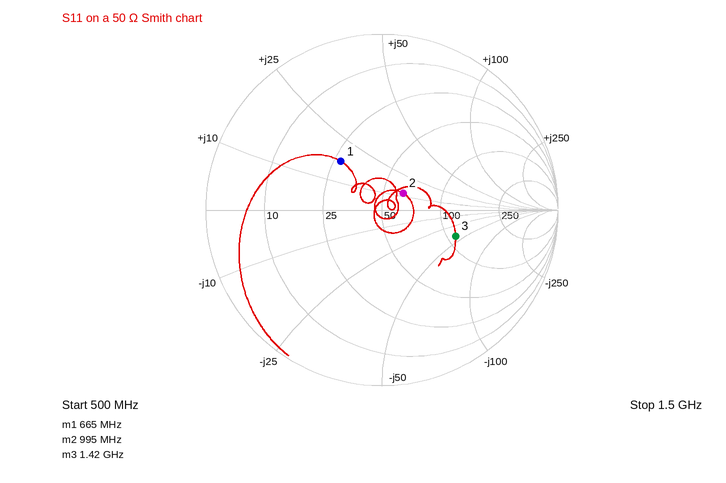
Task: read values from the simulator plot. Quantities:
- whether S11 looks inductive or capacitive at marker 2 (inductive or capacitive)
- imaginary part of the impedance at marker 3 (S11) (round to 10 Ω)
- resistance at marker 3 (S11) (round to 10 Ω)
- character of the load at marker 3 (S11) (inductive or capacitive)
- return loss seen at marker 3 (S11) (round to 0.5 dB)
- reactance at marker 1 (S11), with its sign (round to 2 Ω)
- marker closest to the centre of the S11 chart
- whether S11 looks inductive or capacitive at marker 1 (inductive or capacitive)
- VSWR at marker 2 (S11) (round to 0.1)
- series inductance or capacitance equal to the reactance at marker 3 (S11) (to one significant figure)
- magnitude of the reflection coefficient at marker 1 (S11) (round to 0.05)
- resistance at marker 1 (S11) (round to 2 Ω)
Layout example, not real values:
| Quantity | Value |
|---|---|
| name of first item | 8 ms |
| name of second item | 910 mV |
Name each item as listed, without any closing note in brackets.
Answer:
| Quantity | Value |
|---|---|
| whether S11 looks inductive or capacitive at marker 2 | inductive |
| imaginary part of the impedance at marker 3 (S11) | -40 Ω |
| resistance at marker 3 (S11) | 110 Ω |
| character of the load at marker 3 (S11) | capacitive |
| return loss seen at marker 3 (S11) | 7.0 dB |
| reactance at marker 1 (S11), with its sign | +18 Ω |
| marker closest to the centre of the S11 chart | marker 2 |
| whether S11 looks inductive or capacitive at marker 1 | inductive |
| VSWR at marker 2 (S11) | 1.4 |
| series inductance or capacitance equal to the reactance at marker 3 (S11) | 3 pF |
| magnitude of the reflection coefficient at marker 1 (S11) | 0.35 |
| resistance at marker 1 (S11) | 28 Ω |
